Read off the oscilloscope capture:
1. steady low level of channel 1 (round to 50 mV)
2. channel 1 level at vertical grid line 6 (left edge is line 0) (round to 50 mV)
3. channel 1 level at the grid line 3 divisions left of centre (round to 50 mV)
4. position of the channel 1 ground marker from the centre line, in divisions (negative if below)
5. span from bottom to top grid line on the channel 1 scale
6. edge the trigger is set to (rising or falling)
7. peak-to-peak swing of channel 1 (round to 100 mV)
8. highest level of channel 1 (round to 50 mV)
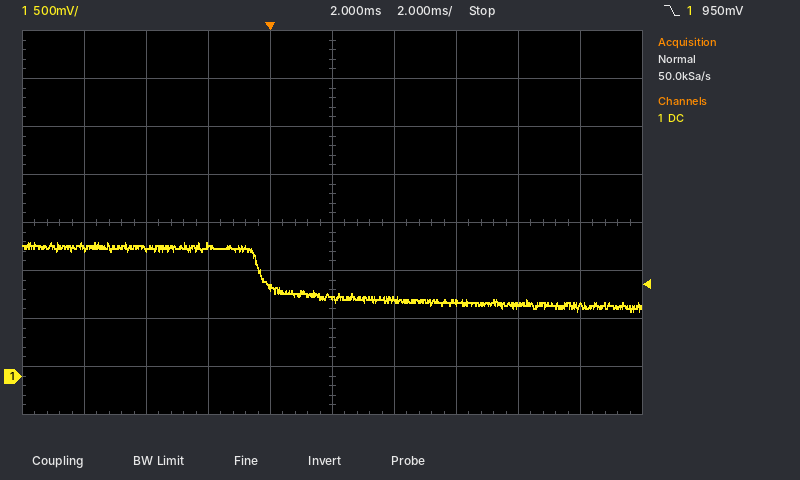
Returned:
750 mV
800 mV
1.35 V
-3.2 div
4 V
falling
700 mV
1.40 V
